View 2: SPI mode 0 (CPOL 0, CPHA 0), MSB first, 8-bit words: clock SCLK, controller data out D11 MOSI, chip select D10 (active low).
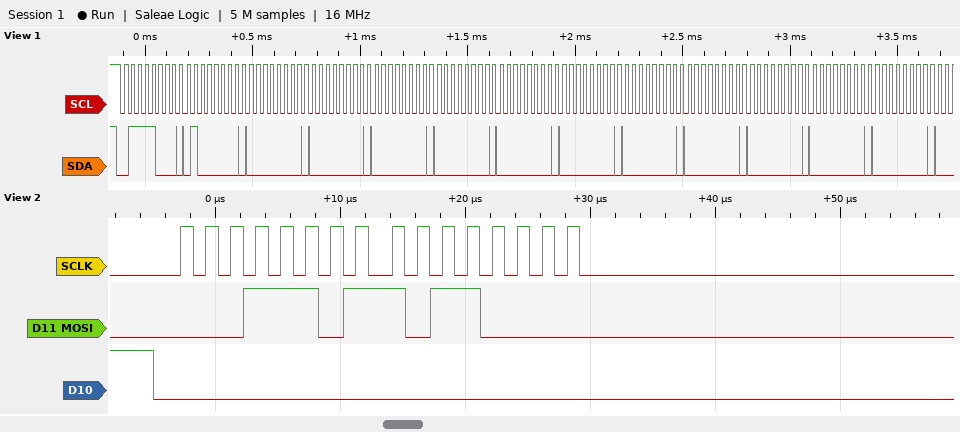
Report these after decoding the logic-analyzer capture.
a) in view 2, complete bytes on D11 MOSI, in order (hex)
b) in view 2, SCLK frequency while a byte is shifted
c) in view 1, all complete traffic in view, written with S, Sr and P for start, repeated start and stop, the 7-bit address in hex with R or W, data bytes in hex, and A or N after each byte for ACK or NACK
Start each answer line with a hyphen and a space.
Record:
- 0x1D 0xB0
- 500 kHz
- S 3CW A 40 A 00 A 00 A 00 A 00 A 00 A 00 A 00 A 00 A 00 A 00 A 00 A
